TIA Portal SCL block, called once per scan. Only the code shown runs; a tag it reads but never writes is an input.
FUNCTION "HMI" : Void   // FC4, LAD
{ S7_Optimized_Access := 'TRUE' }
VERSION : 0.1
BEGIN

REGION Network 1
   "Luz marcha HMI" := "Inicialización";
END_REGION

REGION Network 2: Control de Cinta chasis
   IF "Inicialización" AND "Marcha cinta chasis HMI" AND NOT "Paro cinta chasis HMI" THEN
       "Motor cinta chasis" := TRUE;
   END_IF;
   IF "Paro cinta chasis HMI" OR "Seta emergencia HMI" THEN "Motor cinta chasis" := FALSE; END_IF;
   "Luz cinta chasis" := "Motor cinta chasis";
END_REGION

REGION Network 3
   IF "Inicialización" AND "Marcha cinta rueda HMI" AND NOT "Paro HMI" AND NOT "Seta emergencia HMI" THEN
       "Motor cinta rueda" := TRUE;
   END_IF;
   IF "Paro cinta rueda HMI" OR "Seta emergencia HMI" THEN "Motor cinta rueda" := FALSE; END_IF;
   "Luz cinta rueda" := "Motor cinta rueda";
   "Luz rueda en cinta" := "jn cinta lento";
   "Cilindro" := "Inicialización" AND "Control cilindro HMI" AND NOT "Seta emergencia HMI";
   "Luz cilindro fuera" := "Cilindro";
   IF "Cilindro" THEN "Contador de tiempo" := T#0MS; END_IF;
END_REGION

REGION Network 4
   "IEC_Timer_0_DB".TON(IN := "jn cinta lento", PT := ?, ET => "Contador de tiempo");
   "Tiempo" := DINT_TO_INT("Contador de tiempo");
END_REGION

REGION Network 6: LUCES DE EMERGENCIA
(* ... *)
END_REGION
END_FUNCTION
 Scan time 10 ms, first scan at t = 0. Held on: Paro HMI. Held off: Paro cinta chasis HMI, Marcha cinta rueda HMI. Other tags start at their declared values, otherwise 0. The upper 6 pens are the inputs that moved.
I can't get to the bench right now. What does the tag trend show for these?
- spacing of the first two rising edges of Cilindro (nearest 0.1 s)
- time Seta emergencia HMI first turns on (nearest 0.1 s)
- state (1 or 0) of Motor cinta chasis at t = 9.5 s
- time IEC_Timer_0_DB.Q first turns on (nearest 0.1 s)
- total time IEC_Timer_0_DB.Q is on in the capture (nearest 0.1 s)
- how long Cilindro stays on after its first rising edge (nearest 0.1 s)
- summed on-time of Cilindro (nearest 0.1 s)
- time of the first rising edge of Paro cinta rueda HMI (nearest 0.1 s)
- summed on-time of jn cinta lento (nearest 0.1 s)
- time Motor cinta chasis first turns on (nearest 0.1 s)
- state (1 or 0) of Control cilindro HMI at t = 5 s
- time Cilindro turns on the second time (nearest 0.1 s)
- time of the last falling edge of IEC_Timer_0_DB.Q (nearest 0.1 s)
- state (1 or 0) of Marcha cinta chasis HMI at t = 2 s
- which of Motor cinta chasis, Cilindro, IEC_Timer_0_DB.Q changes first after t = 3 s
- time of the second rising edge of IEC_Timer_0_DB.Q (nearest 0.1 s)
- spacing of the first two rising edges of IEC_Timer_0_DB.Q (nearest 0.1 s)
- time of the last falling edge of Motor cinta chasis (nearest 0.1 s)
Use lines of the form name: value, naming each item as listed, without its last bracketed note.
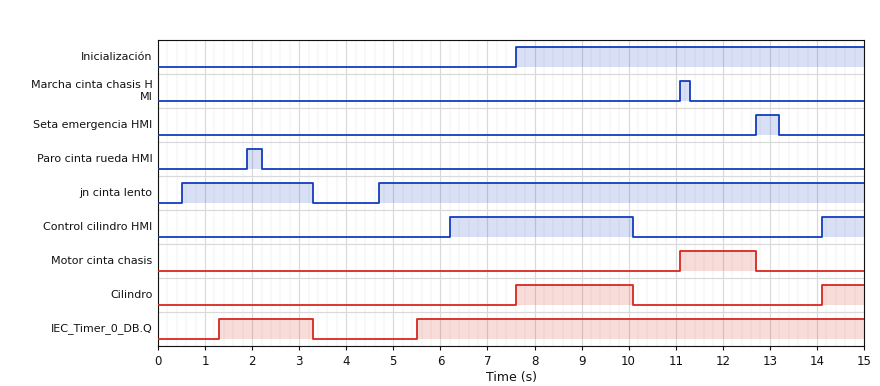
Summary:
spacing of the first two rising edges of Cilindro: 6.5 s
time Seta emergencia HMI first turns on: 12.7 s
state (1 or 0) of Motor cinta chasis at t = 9.5 s: 0
time IEC_Timer_0_DB.Q first turns on: 1.3 s
total time IEC_Timer_0_DB.Q is on in the capture: 11.5 s
how long Cilindro stays on after its first rising edge: 2.5 s
summed on-time of Cilindro: 3.4 s
time of the first rising edge of Paro cinta rueda HMI: 1.9 s
summed on-time of jn cinta lento: 13.1 s
time Motor cinta chasis first turns on: 11.1 s
state (1 or 0) of Control cilindro HMI at t = 5 s: 0
time Cilindro turns on the second time: 14.1 s
time of the last falling edge of IEC_Timer_0_DB.Q: 3.3 s
state (1 or 0) of Marcha cinta chasis HMI at t = 2 s: 0
which of Motor cinta chasis, Cilindro, IEC_Timer_0_DB.Q changes first after t = 3 s: IEC_Timer_0_DB.Q
time of the second rising edge of IEC_Timer_0_DB.Q: 5.5 s
spacing of the first two rising edges of IEC_Timer_0_DB.Q: 4.2 s
time of the last falling edge of Motor cinta chasis: 12.7 s
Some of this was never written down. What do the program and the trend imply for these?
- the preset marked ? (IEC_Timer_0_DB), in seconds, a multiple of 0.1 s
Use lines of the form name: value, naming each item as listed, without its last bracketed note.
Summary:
the preset marked ? (IEC_Timer_0_DB), in seconds, a multiple of 0.1 s: 0.8 s
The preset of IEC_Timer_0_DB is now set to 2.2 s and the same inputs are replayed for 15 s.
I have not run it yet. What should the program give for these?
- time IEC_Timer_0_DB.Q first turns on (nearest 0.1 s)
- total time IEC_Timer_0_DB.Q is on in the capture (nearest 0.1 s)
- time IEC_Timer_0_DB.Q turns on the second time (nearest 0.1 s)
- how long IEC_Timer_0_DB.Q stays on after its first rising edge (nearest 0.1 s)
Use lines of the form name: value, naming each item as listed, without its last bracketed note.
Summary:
time IEC_Timer_0_DB.Q first turns on: 2.7 s
total time IEC_Timer_0_DB.Q is on in the capture: 8.7 s
time IEC_Timer_0_DB.Q turns on the second time: 6.9 s
how long IEC_Timer_0_DB.Q stays on after its first rising edge: 0.6 s
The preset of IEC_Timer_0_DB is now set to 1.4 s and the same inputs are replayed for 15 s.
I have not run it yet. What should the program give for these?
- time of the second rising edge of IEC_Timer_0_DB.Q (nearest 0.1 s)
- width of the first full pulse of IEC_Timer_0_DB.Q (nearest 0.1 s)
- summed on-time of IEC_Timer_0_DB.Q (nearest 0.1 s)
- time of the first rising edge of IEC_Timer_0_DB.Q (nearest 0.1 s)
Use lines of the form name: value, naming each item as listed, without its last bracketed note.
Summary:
time of the second rising edge of IEC_Timer_0_DB.Q: 6.1 s
width of the first full pulse of IEC_Timer_0_DB.Q: 1.4 s
summed on-time of IEC_Timer_0_DB.Q: 10.3 s
time of the first rising edge of IEC_Timer_0_DB.Q: 1.9 s
